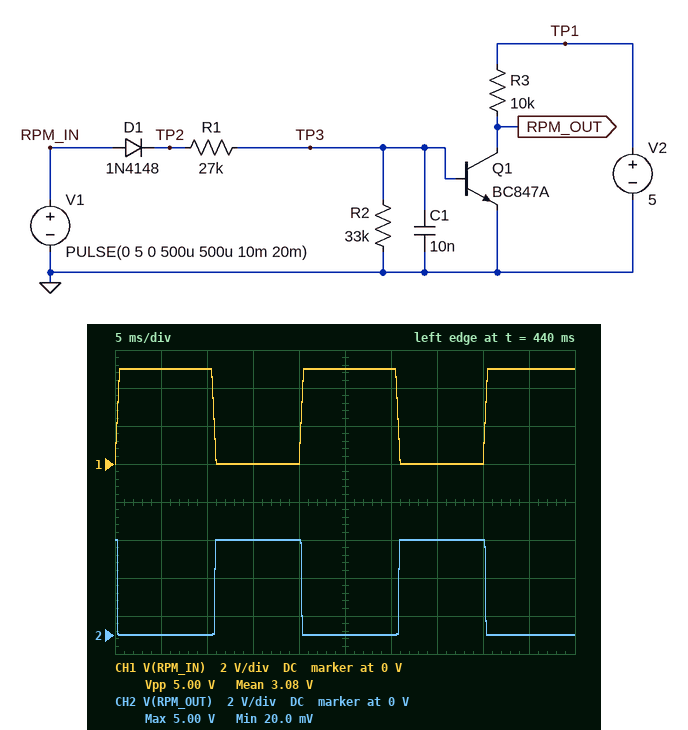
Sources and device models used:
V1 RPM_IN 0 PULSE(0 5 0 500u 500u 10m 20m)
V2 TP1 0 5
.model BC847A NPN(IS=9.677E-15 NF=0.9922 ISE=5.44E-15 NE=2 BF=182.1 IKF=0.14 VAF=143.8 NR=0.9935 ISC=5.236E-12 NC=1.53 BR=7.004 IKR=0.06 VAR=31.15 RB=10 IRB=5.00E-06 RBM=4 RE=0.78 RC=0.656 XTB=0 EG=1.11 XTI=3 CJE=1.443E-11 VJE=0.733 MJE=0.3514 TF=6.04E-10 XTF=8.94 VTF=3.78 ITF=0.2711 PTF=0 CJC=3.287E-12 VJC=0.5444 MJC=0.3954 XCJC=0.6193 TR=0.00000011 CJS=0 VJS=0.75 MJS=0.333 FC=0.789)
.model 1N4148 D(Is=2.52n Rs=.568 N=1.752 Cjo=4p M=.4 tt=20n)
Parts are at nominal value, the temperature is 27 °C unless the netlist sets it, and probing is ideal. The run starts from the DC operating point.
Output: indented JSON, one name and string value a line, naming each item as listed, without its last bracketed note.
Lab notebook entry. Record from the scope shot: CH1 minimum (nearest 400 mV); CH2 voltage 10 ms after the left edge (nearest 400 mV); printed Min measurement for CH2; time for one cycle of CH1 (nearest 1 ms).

{
  "CH1 minimum": "0 V",
  "CH2 voltage 10 ms after the left edge": "0 V",
  "printed Min measurement for CH2": "20.0 mV",
  "time for one cycle of CH1": "20 ms"
}
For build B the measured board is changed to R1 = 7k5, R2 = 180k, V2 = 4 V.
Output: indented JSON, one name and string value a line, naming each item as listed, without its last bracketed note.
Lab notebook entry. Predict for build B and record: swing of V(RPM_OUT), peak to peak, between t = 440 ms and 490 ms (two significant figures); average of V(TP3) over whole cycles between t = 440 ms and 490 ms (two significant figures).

{
  "swing of V(RPM_OUT), peak to peak, between t = 440 ms and 490 ms": "4.0 V",
  "average of V(TP3) over whole cycles between t = 440 ms and 490 ms": "420 mV"
}
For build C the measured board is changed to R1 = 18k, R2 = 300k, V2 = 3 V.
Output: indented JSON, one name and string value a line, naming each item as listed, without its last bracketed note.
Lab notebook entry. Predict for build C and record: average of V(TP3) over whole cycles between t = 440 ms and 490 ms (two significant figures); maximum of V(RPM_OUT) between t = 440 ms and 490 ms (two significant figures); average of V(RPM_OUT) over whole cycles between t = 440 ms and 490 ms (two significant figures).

{
  "average of V(TP3) over whole cycles between t = 440 ms and 490 ms": "440 mV",
  "maximum of V(RPM_OUT) between t = 440 ms and 490 ms": "3.0 V",
  "average of V(RPM_OUT) over whole cycles between t = 440 ms and 490 ms": "1.4 V"
}
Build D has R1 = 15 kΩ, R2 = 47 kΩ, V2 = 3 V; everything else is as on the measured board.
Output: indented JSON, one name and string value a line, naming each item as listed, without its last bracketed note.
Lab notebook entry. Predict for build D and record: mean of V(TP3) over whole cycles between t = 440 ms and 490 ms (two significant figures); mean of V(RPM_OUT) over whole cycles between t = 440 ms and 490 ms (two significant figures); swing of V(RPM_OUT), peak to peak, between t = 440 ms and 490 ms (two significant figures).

{
  "mean of V(TP3) over whole cycles between t = 440 ms and 490 ms": "370 mV",
  "mean of V(RPM_OUT) over whole cycles between t = 440 ms and 490 ms": "1.4 V",
  "swing of V(RPM_OUT), peak to peak, between t = 440 ms and 490 ms": "3.0 V"
}
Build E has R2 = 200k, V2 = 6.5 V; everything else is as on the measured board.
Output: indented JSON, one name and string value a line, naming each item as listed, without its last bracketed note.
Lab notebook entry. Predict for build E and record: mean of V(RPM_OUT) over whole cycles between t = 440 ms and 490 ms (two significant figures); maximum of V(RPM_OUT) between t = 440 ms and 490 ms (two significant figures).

{
  "mean of V(RPM_OUT) over whole cycles between t = 440 ms and 490 ms": "3.0 V",
  "maximum of V(RPM_OUT) between t = 440 ms and 490 ms": "6.5 V"
}
